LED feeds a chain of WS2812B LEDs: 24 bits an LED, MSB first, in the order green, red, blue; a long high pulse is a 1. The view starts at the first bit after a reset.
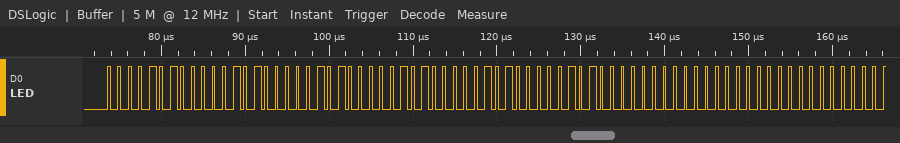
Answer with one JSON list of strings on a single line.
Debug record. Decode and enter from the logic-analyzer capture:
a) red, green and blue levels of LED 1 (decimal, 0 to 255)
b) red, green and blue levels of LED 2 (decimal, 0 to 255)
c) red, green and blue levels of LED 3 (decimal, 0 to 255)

["10, 10, 10", "10, 10, 10", "0, 0, 0"]
